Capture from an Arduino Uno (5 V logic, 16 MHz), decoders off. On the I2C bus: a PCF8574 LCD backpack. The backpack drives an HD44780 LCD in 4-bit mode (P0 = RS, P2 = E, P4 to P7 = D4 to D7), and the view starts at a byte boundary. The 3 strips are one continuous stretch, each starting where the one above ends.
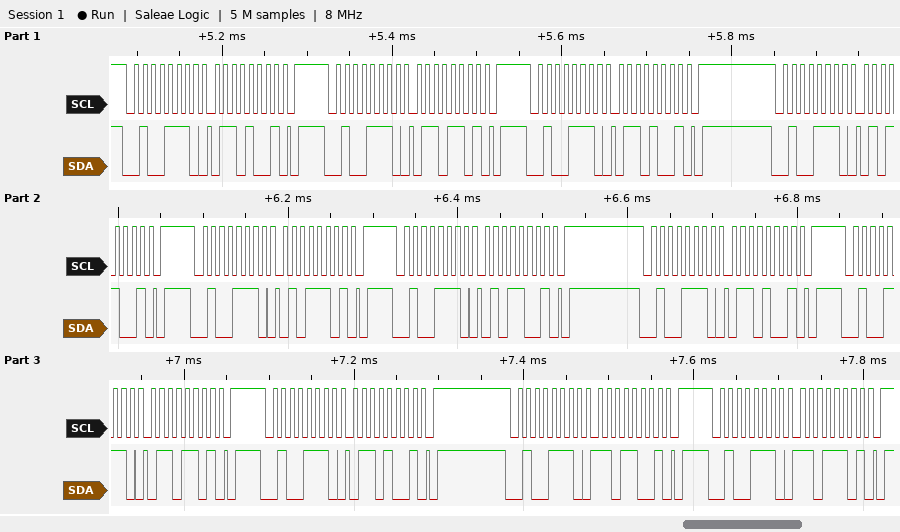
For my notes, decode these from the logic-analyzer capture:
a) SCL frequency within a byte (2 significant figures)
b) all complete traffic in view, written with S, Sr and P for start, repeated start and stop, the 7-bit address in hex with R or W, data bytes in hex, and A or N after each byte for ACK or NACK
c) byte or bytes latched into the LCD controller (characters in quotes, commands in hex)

100 kHz
S 27W A 69 A P S 27W A 6D A P S 27W A 69 A P S 27W A 59 A P S 27W A 5D A P S 27W A 59 A P S 27W A 69 A P S 27W A 6D A P S 27W A 69 A P S 27W A D9 A P S 27W A DD A P
'e'
